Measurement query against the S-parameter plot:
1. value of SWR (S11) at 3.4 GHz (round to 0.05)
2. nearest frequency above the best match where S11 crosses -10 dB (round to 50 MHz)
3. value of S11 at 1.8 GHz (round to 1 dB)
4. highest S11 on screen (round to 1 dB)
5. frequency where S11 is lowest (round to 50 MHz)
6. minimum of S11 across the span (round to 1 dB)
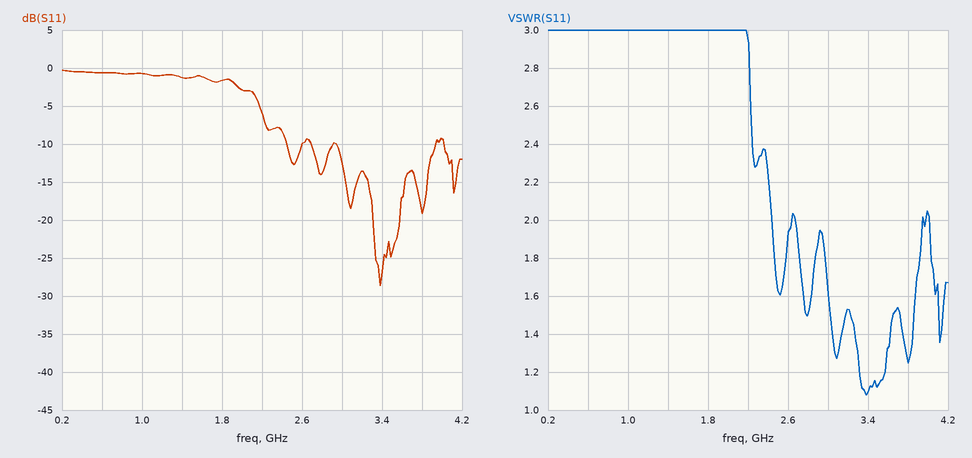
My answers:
1.10
3.95 GHz
-2 dB
0 dB
3.40 GHz
-29 dB
